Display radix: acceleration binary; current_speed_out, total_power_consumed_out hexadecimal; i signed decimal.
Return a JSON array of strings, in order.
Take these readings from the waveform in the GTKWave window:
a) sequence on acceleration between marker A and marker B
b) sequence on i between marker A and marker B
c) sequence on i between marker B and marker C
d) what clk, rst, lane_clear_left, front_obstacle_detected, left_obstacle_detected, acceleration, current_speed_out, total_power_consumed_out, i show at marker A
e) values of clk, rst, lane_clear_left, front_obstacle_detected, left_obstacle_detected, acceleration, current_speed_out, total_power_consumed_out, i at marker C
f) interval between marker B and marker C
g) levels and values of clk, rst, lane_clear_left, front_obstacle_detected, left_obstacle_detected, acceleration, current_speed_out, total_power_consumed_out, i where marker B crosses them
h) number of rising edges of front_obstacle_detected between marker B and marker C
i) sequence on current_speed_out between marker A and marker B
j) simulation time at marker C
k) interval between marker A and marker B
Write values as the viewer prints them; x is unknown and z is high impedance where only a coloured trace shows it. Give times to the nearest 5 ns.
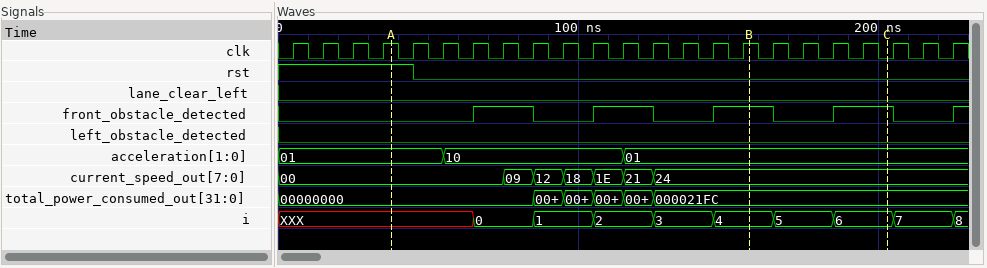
["01, 10, 01", "XXX, 0, 1, 2, 3, 4", "4, 5, 6", "clk=1, rst=1, lane_clear_left=0, front_obstacle_detected=0, left_obstacle_detected=0, acceleration=01, current_speed_out=00, total_power_consumed_out=00000000, i=XXX", "clk=0, rst=0, lane_clear_left=0, front_obstacle_detected=1, left_obstacle_detected=0, acceleration=01, current_speed_out=24, total_power_consumed_out=000021FC, i=6", "45 ns", "clk=1, rst=0, lane_clear_left=0, front_obstacle_detected=1, left_obstacle_detected=0, acceleration=01, current_speed_out=24, total_power_consumed_out=000021FC, i=4", "1", "00, 09, 12, 18, 1E, 21, 24", "205 ns", "120 ns"]
